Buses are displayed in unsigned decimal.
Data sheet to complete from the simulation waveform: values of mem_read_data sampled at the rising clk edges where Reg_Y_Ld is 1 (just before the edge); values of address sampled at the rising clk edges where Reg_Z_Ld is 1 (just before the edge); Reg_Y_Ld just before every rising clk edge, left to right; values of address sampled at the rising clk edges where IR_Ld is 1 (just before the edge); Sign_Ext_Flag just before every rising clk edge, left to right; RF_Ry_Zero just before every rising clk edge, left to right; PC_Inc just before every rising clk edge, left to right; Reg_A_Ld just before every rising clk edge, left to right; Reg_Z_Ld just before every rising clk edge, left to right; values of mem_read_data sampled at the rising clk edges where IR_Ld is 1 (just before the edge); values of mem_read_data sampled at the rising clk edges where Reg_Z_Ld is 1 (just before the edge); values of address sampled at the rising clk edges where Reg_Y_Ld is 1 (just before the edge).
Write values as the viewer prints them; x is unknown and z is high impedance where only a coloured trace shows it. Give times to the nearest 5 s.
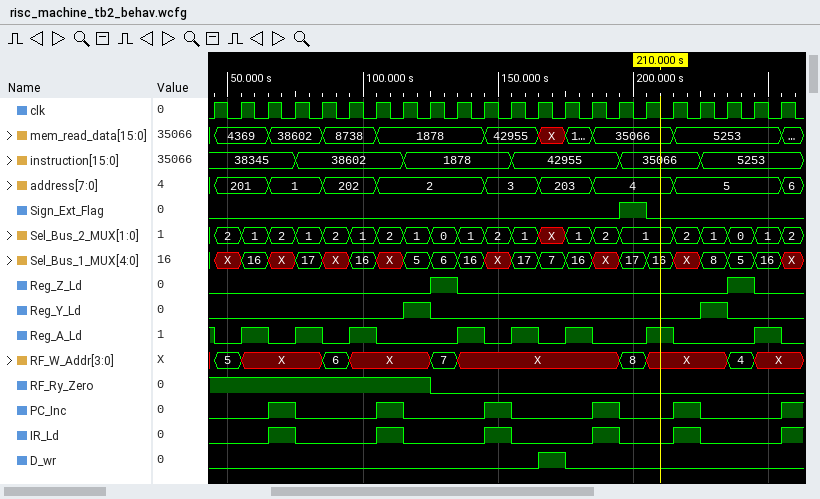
1878, 5253
2, 5
0 0 0 0 0 0 0 0 1 0 0 0 0 0 0 0 0 0 0 1 0 0
1, 2, 3, 4, 5
0 0 0 0 0 0 0 0 0 0 0 0 0 0 0 0 1 0 0 0 0 0
1 1 1 1 1 1 1 1 1 0 0 0 0 0 0 0 0 0 0 0 0 0
0 0 0 1 0 0 0 1 0 0 0 1 0 0 0 1 0 0 1 0 0 0
1 0 1 0 1 0 1 0 0 0 1 0 1 0 1 0 0 1 0 0 0 1
0 0 0 0 0 0 0 0 0 1 0 0 0 0 0 0 0 0 0 0 1 0
38602, 1878, 42955, 35066, 5253
1878, 5253
2, 5
